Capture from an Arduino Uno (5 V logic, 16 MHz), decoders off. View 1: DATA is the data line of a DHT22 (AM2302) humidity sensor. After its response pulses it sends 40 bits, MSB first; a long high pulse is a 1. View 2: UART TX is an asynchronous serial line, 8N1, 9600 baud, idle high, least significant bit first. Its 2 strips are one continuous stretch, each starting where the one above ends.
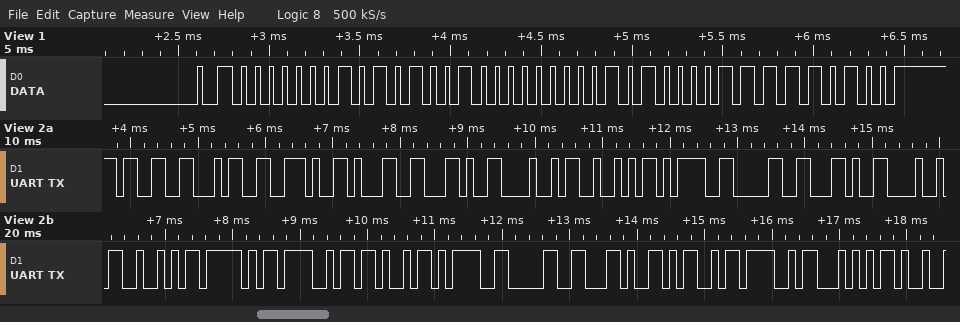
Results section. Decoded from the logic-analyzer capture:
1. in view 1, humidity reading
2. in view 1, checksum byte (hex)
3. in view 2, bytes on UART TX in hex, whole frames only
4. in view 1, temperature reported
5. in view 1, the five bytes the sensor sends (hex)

33.8 %
0xF4
0x33 0x34 0x2E 0x31 0x2C 0x48 0x52 0x3D 0x30 0x2C 0x48 0x52 0x5F 0x4F 0x4B 0x3D 0x30 0x2C 0x4D 0x4F 0x54
16.1 °C
01 52 00 A1 F4
